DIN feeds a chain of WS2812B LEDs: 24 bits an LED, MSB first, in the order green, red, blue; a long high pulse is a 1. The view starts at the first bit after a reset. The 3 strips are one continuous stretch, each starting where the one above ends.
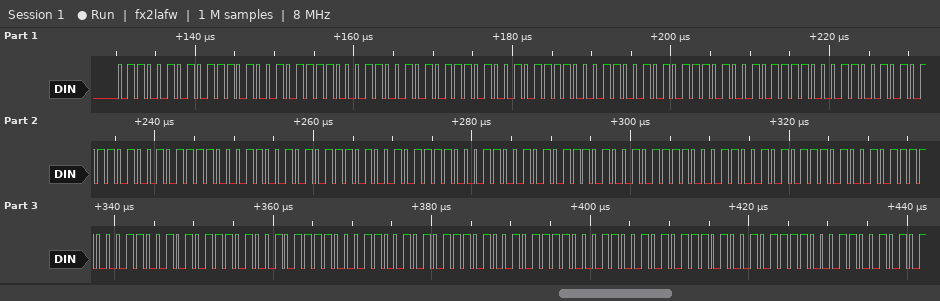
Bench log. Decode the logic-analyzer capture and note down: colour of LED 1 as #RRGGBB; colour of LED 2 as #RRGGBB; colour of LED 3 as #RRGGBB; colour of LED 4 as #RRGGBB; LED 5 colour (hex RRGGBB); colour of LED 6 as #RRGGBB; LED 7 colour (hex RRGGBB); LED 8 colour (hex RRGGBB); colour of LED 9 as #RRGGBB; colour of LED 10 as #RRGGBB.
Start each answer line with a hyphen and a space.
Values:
- #7465BC
- #7465BC
- #7465BC
- #7465BC
- #7465BC
- #7465BC
- #7465BC
- #7465BC
- #7465BC
- #7465BC
